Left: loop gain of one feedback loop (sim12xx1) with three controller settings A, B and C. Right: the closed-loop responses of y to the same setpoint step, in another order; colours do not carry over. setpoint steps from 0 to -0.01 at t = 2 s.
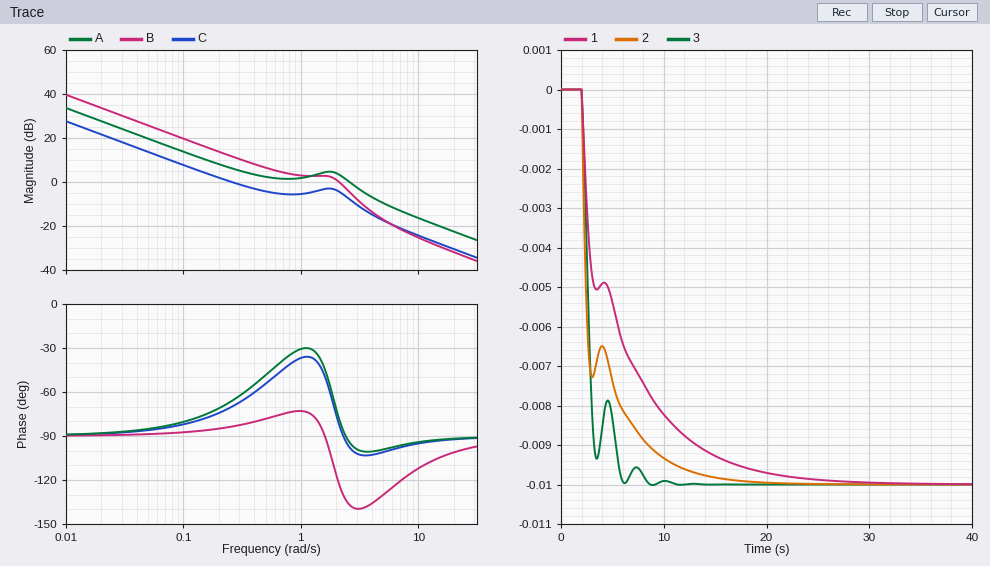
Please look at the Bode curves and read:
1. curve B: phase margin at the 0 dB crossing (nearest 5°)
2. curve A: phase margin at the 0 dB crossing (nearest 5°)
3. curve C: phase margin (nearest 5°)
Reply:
55°
85°
110°
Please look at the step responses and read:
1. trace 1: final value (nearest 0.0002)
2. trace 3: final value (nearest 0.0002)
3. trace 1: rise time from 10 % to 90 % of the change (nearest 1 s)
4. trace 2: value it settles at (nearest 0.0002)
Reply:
-0.0100
-0.0100
11 s
-0.0100
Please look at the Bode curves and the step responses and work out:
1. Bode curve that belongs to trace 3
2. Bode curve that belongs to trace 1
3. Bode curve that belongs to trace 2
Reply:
B
C
A
